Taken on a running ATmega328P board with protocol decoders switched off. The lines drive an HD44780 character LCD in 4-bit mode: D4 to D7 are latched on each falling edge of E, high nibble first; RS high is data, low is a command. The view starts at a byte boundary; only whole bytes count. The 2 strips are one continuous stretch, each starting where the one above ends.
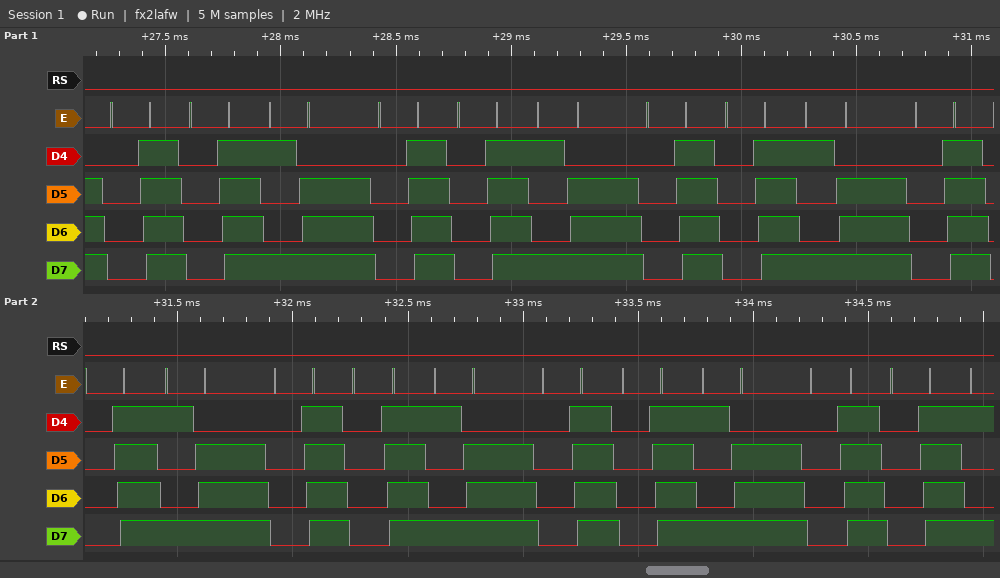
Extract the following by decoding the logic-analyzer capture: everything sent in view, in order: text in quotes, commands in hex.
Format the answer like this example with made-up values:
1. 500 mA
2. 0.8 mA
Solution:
1. 0x0F 0x0F 0x9E 0x0F 0x0F 0x9E 0x0F 0x0F 0x9E 0x0F 0x0F 0x9E 0x0F 0x0F 0x9E 0x0F 0x0F 0x9E 0x0F 0x0F
